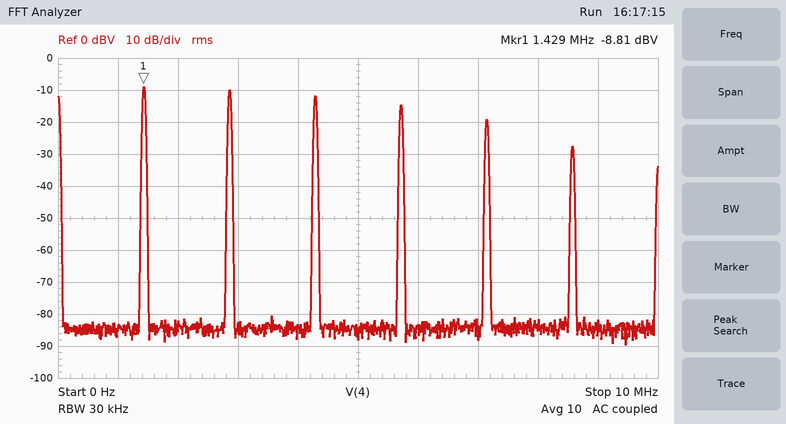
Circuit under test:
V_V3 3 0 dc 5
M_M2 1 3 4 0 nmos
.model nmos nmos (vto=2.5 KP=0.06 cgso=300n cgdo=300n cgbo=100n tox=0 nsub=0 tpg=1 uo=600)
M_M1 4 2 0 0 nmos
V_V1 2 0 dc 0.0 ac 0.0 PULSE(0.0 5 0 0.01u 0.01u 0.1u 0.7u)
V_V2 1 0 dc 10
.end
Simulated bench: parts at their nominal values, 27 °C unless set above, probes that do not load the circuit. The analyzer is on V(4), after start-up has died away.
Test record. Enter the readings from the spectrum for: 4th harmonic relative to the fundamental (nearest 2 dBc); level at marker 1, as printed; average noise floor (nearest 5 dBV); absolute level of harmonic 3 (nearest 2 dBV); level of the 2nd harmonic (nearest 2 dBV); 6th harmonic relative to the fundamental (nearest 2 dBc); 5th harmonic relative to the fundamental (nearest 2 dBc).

-6 dBc
-8.81 dBV
-85 dBV
-12 dBV
-10 dBV
-18 dBc
-10 dBc
